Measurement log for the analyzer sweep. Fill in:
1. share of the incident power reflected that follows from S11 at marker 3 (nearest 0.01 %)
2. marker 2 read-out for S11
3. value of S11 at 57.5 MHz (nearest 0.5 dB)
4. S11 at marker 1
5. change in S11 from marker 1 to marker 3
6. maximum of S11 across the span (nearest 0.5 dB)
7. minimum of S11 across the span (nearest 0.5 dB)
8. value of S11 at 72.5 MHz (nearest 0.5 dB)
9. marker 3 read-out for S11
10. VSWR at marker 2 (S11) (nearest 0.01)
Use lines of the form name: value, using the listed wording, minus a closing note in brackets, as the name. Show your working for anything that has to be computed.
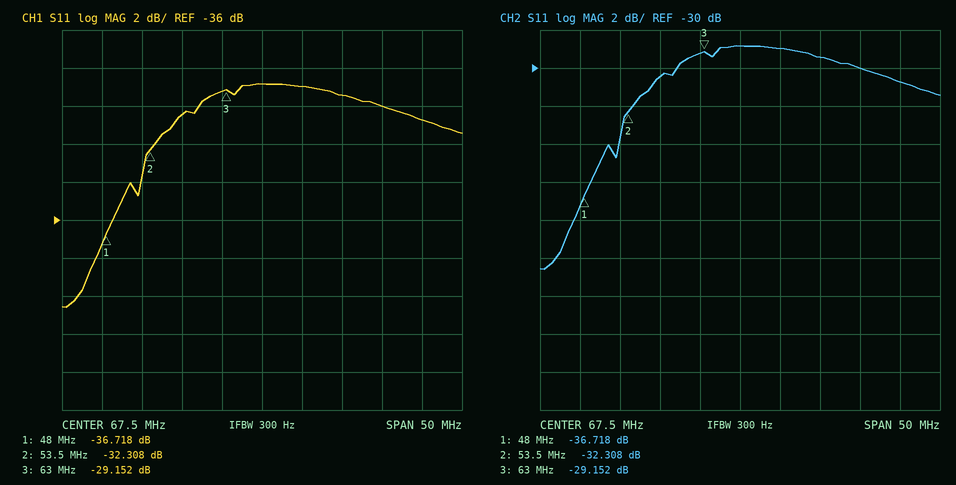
share of the incident power reflected that follows from S11 at marker 3: 10^(-29.152/10) ≈ 0.12 %
marker 2 read-out for S11: -32.308 dB
value of S11 at 57.5 MHz: -30.5 dB
S11 at marker 1: -36.718 dB
change in S11 from marker 1 to marker 3: -29.152 − (-36.718) = 7.566 dB
maximum of S11 across the span: -29.0 dB
minimum of S11 across the span: -40.5 dB
value of S11 at 72.5 MHz: -29.0 dB
marker 3 read-out for S11: -29.152 dB
VSWR at marker 2 (S11): (1 + 0.0242)/(1 − 0.0242) ≈ 1.05
